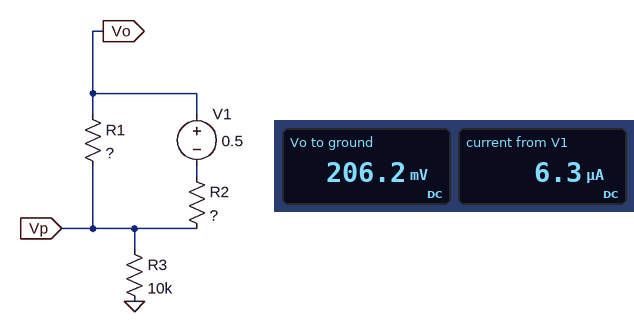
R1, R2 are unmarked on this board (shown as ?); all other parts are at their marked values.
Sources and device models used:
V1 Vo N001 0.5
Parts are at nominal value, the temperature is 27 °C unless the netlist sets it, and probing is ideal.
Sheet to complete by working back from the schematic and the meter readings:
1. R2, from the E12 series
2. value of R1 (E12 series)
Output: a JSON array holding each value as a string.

["47 kΩ", "33 kΩ"]
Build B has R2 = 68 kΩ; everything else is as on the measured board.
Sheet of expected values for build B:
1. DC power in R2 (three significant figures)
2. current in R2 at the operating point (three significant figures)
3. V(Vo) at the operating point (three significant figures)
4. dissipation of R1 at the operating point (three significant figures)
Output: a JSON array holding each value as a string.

["1.67 µW", "4.95 µA", "163 mV", "809 nW"]
